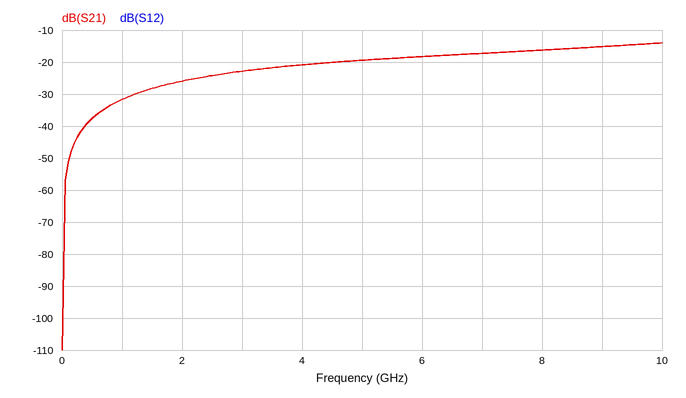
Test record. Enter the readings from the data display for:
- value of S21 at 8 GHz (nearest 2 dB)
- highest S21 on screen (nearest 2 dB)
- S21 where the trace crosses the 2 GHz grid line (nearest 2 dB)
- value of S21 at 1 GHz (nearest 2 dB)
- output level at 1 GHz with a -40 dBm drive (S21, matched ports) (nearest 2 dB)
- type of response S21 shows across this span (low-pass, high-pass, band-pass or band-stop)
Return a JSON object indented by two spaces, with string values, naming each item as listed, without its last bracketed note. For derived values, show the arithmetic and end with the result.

{
  "value of S21 at 8 GHz": "-16 dB",
  "highest S21 on screen": "-14 dB",
  "S21 where the trace crosses the 2 GHz grid line": "-26 dB",
  "value of S21 at 1 GHz": "-32 dB",
  "output level at 1 GHz with a -40 dBm drive (S21, matched ports)": "-40 dBm + (-32 dB) = -72 dBm",
  "type of response S21 shows across this span": "high-pass"
}
